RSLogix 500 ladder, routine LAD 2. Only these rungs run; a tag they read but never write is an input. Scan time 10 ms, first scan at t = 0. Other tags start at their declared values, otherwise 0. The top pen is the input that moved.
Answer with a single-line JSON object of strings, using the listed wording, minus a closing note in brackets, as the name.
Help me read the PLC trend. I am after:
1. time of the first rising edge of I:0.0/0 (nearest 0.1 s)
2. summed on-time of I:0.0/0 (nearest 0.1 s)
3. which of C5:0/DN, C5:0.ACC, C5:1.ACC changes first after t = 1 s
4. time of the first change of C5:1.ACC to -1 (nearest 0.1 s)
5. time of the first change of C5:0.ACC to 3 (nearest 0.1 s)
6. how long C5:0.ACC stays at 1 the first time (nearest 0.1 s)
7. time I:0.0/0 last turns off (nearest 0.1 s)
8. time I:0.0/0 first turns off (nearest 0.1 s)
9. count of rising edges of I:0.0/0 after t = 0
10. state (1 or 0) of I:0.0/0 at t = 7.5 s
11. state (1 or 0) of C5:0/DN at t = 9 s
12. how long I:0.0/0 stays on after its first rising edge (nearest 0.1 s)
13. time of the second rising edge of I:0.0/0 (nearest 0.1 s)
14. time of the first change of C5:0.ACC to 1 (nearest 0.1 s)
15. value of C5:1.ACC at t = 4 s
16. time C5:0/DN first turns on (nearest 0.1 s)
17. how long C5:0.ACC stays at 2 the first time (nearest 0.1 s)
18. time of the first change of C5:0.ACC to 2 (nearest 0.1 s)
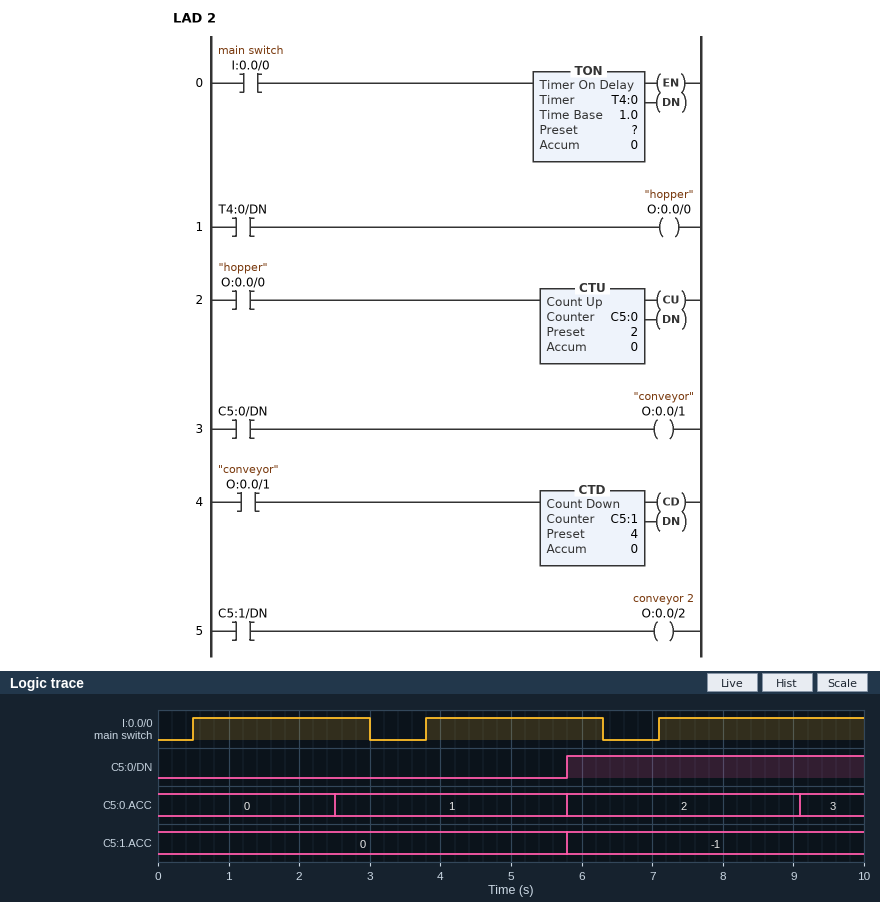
{"time of the first rising edge of I:0.0/0": "0.5 s", "summed on-time of I:0.0/0": "7.9 s", "which of C5:0/DN, C5:0.ACC, C5:1.ACC changes first after t = 1 s": "C5:0.ACC", "time of the first change of C5:1.ACC to -1": "5.8 s", "time of the first change of C5:0.ACC to 3": "9.1 s", "how long C5:0.ACC stays at 1 the first time": "3.3 s", "time I:0.0/0 last turns off": "6.3 s", "time I:0.0/0 first turns off": "3.0 s", "count of rising edges of I:0.0/0 after t = 0": "3", "state (1 or 0) of I:0.0/0 at t = 7.5 s": "1", "state (1 or 0) of C5:0/DN at t = 9 s": "1", "how long I:0.0/0 stays on after its first rising edge": "2.5 s", "time of the second rising edge of I:0.0/0": "3.8 s", "time of the first change of C5:0.ACC to 1": "2.5 s", "value of C5:1.ACC at t = 4 s": "0", "time C5:0/DN first turns on": "5.8 s", "how long C5:0.ACC stays at 2 the first time": "3.3 s", "time of the first change of C5:0.ACC to 2": "5.8 s"}
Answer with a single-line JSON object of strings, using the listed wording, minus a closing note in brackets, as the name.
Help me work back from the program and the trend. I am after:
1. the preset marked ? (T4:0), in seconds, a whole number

{"the preset marked ? (T4:0), in seconds, a whole number": "2 s"}
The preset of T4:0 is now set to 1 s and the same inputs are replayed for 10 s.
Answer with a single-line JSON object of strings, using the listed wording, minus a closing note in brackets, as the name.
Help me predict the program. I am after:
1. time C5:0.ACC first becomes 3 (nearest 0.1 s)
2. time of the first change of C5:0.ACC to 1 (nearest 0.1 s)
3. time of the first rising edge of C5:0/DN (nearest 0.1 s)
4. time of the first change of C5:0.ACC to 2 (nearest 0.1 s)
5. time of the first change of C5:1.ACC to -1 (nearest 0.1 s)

{"time C5:0.ACC first becomes 3": "8.1 s", "time of the first change of C5:0.ACC to 1": "1.5 s", "time of the first rising edge of C5:0/DN": "4.8 s", "time of the first change of C5:0.ACC to 2": "4.8 s", "time of the first change of C5:1.ACC to -1": "4.8 s"}
